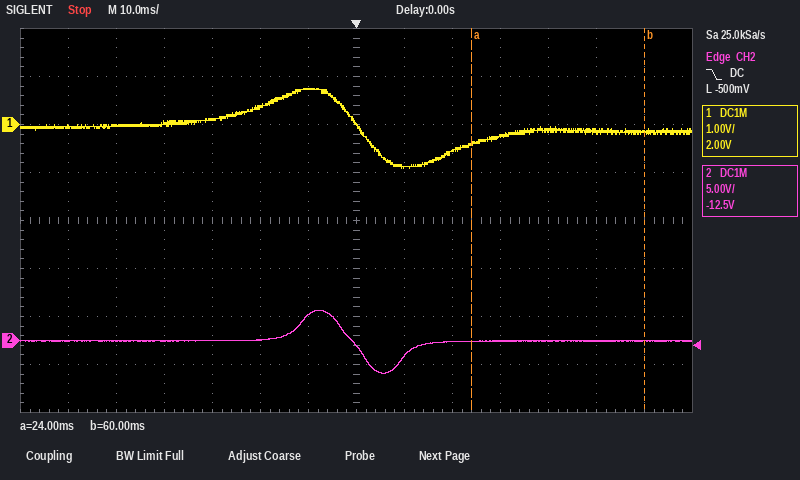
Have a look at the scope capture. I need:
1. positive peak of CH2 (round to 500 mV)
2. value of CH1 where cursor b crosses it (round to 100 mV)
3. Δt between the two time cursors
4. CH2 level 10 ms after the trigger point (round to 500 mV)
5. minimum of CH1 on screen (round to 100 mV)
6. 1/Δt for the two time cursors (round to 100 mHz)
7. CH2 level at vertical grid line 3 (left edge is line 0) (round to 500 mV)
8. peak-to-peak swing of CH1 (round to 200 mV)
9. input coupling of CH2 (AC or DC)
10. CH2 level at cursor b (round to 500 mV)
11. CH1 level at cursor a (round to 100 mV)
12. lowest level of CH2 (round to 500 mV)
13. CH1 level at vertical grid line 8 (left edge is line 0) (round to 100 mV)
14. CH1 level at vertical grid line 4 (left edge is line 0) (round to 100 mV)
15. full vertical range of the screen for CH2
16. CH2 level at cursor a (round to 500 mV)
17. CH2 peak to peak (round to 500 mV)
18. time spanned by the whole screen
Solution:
3.0 V
-200 mV
36 ms
-1.5 V
-900 mV
27.8 Hz
0.0 V
1.6 V
DC
0.0 V
-400 mV
-3.5 V
-900 mV
100 mV
40 V
0.0 V
6.5 V
140 ms
